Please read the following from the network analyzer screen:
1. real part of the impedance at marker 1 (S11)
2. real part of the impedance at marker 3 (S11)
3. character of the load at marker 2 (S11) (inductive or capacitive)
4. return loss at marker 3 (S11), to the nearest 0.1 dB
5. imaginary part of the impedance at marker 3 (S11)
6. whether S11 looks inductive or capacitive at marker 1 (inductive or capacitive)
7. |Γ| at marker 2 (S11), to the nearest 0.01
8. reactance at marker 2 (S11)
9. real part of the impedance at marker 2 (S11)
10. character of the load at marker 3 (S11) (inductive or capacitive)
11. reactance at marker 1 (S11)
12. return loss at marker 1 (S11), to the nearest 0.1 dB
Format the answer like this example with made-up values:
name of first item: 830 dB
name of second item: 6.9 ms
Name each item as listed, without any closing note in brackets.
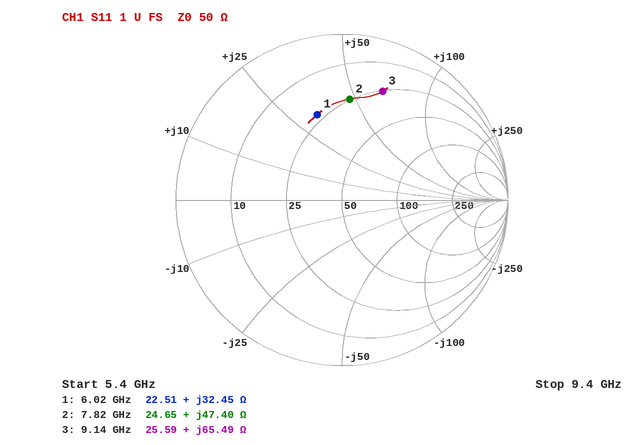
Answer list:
real part of the impedance at marker 1: 22.51 Ω
real part of the impedance at marker 3: 25.59 Ω
character of the load at marker 2 (S11): inductive
return loss at marker 3 (S11), to the nearest 0.1 dB: 3.1 dB
imaginary part of the impedance at marker 3: +65.49 Ω
whether S11 looks inductive or capacitive at marker 1: inductive
|Γ| at marker 2 (S11), to the nearest 0.01: 0.61
reactance at marker 2: +47.40 Ω
real part of the impedance at marker 2: 24.65 Ω
character of the load at marker 3 (S11): inductive
reactance at marker 1: +32.45 Ω
return loss at marker 1 (S11), to the nearest 0.1 dB: 5.4 dB
